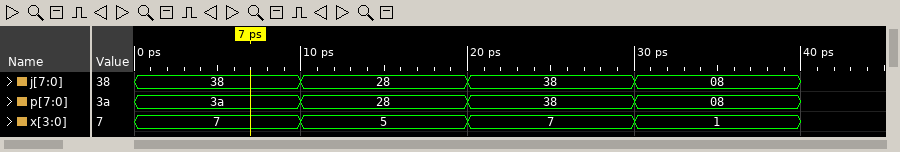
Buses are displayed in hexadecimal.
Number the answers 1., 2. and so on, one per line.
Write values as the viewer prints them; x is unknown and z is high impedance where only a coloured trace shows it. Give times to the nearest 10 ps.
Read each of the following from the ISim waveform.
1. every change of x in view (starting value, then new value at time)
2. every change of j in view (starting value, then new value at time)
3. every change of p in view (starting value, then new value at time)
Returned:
1. 7, 5 at 10 ps, 7 at 20 ps, 1 at 30 ps
2. 38, 28 at 10 ps, 38 at 20 ps, 08 at 30 ps
3. 3a, 28 at 10 ps, 38 at 20 ps, 08 at 30 ps
